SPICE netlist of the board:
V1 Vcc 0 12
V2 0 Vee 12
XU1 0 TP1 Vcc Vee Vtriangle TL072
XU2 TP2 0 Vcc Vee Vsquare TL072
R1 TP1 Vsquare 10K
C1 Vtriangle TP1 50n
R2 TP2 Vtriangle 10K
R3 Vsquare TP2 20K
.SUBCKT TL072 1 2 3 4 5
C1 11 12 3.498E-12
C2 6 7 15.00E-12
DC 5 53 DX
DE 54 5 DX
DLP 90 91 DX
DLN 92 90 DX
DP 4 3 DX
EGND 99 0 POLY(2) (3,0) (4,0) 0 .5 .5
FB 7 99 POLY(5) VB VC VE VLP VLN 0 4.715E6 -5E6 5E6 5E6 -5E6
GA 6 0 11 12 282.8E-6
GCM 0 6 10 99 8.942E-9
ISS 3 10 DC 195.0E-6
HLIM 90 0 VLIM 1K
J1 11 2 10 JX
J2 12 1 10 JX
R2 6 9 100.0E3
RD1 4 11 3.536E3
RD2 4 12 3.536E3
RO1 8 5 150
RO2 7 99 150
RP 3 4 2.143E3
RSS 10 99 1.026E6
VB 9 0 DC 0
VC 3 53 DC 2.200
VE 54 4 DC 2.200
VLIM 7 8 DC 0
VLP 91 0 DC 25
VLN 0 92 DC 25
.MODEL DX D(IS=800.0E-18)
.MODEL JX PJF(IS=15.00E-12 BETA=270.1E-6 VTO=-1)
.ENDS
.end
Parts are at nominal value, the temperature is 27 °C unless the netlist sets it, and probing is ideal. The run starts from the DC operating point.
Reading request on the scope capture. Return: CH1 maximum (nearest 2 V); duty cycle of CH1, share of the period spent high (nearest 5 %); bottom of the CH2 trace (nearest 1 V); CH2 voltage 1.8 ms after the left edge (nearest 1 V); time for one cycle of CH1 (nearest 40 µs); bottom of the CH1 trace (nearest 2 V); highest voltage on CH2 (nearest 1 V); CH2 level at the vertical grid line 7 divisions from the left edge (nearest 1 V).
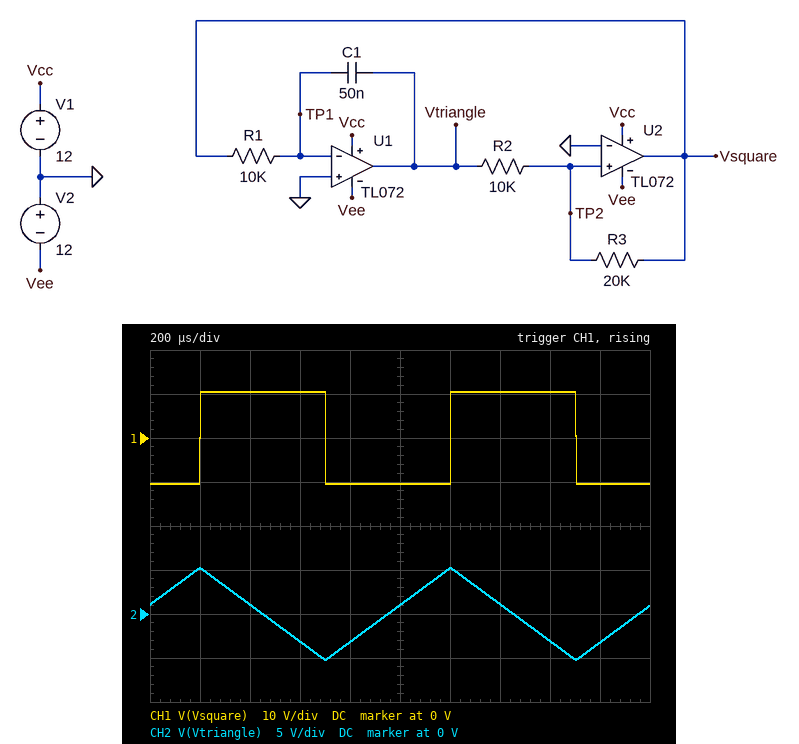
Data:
10 V
50 %
-5 V
-3 V
1.00 ms
-10 V
5 V
1 V
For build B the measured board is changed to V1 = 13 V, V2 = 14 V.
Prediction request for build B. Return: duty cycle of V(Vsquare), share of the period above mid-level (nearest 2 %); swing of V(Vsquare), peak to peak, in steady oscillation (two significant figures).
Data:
52 %
24 V
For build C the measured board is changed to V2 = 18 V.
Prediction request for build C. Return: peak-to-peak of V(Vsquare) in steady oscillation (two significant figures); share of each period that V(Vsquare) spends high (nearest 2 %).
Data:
27 V
62 %
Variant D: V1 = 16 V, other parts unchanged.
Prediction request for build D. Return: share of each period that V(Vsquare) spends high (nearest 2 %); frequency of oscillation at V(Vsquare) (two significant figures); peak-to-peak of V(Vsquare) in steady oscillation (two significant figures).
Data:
42 %
970 Hz
25 V
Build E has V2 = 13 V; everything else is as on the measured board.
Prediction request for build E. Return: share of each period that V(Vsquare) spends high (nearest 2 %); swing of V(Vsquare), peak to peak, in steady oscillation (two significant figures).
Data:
52 %
22 V
